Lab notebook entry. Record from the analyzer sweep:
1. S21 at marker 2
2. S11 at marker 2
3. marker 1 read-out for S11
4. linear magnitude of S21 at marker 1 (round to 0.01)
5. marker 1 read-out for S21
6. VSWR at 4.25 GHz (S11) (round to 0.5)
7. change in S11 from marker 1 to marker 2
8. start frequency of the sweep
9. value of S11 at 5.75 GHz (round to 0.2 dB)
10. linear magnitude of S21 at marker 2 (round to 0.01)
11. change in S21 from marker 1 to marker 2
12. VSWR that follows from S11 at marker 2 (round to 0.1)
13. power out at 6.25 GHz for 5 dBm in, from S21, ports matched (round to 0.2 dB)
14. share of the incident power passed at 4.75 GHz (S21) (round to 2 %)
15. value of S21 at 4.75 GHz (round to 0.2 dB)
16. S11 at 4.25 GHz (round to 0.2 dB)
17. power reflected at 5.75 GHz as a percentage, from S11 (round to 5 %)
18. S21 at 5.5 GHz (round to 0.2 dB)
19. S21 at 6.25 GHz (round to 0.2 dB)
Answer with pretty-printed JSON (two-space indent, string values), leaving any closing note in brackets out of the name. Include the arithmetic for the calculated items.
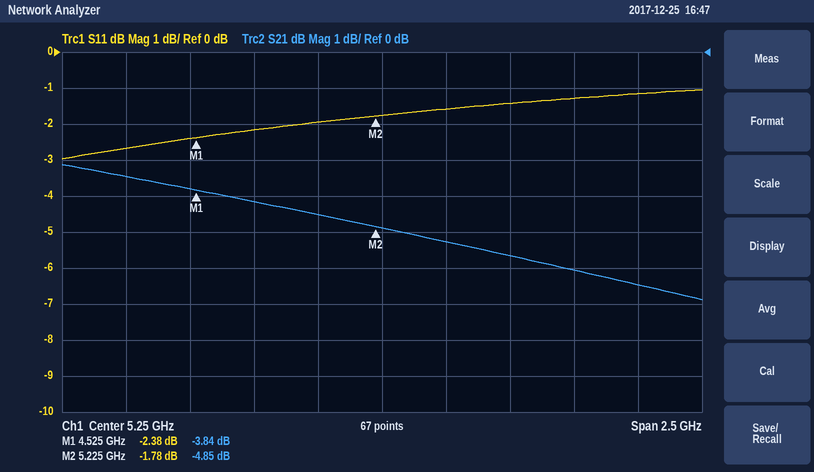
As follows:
{
  "S21 at marker 2": "-4.85 dB",
  "S11 at marker 2": "-1.78 dB",
  "marker 1 read-out for S11": "-2.38 dB",
  "linear magnitude of S21 at marker 1": "10^(-3.84/20) ≈ 0.64",
  "marker 1 read-out for S21": "-3.84 dB",
  "VSWR at 4.25 GHz (S11)": "|Γ| = 10^(-2.6/20) = 0.7413; VSWR = (1 + 0.7413)/(1 − 0.7413) ≈ 6.73, so 6.5 to the nearest 0.5",
  "change in S11 from marker 1 to marker 2": "-1.78 − (-2.38) = 0.60 dB",
  "start frequency of the sweep": "4 GHz",
  "value of S11 at 5.75 GHz": "-1.4 dB",
  "linear magnitude of S21 at marker 2": "10^(-4.85/20) ≈ 0.57",
  "change in S21 from marker 1 to marker 2": "-4.85 − (-3.84) = -1.01 dB",
  "VSWR that follows from S11 at marker 2": "(1 + 0.8147)/(1 − 0.8147) ≈ 9.8",
  "power out at 6.25 GHz for 5 dBm in, from S21, ports matched": "5 dBm + (-6.4 dB) = -1.4 dBm",
  "share of the incident power passed at 4.75 GHz (S21)": "10^(-4.2/10) ≈ 38 %",
  "value of S21 at 4.75 GHz": "-4.2 dB",
  "S11 at 4.25 GHz": "-2.6 dB",
  "power reflected at 5.75 GHz as a percentage, from S11": "10^(-1.4/10) ≈ 72.4 %, so 70 % to the nearest 5 %",
  "S21 at 5.5 GHz": "-5.2 dB",
  "S21 at 6.25 GHz": "-6.4 dB"
}
